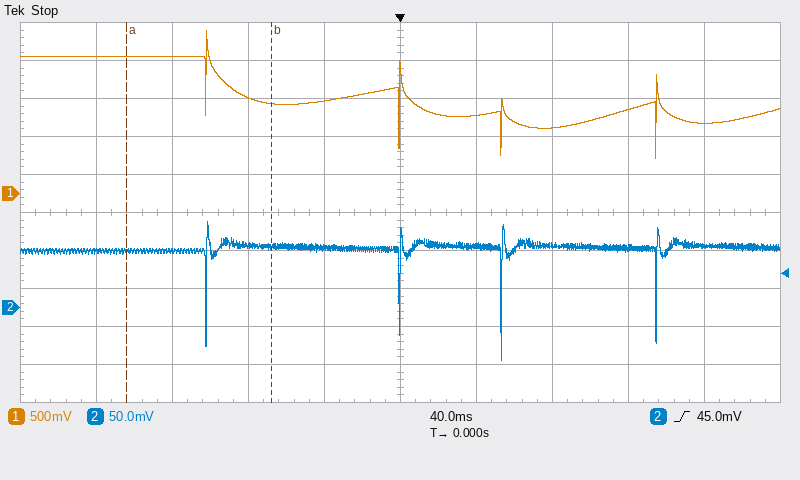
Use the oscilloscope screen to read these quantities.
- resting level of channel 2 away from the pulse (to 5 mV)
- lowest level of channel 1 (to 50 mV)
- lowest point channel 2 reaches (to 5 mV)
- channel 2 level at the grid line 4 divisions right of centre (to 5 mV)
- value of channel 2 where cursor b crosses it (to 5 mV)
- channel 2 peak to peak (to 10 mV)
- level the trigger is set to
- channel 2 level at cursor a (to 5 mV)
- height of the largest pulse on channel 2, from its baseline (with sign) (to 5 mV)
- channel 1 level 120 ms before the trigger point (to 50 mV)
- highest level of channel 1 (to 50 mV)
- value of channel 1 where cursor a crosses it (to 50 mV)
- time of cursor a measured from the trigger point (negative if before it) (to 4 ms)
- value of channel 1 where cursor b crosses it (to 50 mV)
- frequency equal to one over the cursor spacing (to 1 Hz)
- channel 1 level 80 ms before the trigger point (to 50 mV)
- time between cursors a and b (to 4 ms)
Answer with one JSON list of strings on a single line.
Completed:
["80 mV", "450 mV", "-70 mV", "80 mV", "80 mV", "180 mV", "45.0 mV", "75 mV", "-150 mV", "1.80 V", "2.15 V", "1.80 V", "-144 ms", "1.20 V", "13 Hz", "1.25 V", "76 ms"]
